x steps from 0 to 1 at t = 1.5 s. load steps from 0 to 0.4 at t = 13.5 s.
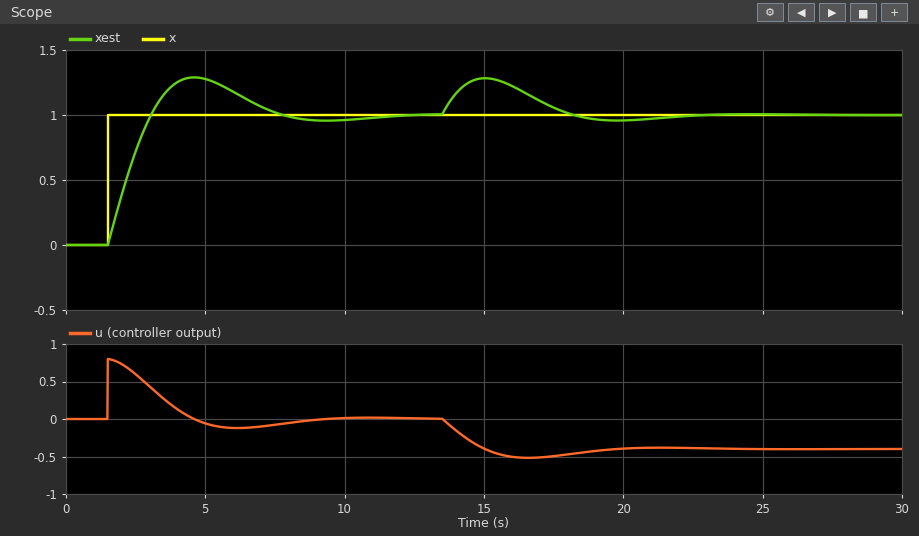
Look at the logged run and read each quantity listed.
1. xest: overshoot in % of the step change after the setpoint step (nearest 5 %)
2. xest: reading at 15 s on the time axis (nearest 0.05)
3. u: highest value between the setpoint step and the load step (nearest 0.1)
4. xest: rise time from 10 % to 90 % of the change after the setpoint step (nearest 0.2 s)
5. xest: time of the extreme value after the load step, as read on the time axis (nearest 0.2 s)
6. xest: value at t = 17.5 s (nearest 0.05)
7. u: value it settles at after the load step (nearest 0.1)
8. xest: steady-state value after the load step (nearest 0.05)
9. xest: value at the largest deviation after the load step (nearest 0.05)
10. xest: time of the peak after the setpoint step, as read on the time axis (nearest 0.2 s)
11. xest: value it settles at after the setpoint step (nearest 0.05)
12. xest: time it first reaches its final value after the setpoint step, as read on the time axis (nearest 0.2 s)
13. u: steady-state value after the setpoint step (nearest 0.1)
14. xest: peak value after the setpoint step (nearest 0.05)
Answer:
30 %
1.30
0.8
1.2 s
15.0 s
1.05
-0.4
1.00
1.30
4.6 s
1.00
3.0 s
0.0
1.30
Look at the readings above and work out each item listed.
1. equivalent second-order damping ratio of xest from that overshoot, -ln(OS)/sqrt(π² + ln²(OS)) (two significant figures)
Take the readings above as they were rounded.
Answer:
0.36
